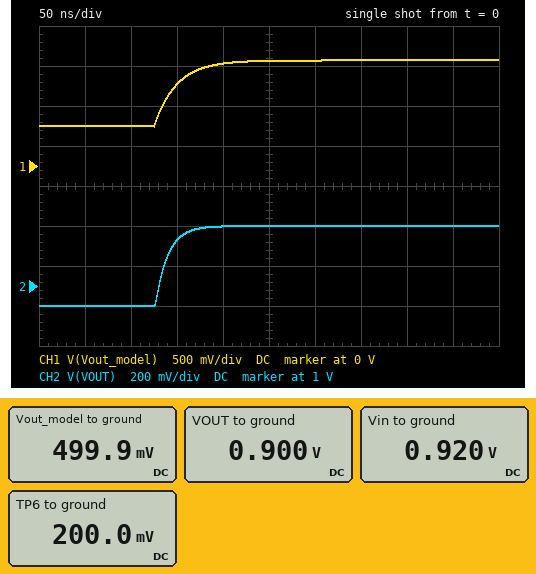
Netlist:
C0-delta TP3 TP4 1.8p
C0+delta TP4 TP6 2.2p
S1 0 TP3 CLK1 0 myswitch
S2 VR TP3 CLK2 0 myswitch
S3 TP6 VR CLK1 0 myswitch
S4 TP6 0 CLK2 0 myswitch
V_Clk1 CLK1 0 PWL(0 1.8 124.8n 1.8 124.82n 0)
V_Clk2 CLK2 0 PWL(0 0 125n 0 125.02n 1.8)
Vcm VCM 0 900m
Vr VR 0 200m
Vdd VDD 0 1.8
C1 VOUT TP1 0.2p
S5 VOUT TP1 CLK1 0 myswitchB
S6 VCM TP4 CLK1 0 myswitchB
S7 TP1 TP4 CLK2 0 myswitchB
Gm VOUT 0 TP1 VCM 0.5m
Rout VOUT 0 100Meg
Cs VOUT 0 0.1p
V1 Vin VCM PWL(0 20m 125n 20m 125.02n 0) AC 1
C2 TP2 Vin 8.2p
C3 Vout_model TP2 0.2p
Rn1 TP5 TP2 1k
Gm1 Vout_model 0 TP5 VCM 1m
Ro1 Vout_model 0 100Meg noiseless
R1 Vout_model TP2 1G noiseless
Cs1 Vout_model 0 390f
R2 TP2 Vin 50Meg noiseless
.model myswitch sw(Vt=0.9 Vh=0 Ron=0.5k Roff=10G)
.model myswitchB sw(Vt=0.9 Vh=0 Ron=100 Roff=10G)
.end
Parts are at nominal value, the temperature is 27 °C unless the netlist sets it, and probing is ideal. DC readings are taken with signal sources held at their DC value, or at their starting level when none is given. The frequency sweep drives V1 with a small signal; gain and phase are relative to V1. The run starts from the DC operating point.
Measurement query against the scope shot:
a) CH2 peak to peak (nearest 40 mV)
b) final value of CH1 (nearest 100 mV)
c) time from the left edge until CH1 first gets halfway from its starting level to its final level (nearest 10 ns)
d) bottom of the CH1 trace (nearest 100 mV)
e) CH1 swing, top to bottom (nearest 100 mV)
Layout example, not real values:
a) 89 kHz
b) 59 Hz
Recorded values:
a) 400 mV
b) 1.3 V
c) 140 ns
d) 500 mV
e) 800 mV
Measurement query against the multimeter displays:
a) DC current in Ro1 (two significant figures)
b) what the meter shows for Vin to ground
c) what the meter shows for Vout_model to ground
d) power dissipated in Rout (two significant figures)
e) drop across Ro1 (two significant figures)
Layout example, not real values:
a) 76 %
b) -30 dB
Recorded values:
a) 5.0 nA
b) 0.920 V
c) 499.9 mV
d) 8.1 nW
e) 500 mV
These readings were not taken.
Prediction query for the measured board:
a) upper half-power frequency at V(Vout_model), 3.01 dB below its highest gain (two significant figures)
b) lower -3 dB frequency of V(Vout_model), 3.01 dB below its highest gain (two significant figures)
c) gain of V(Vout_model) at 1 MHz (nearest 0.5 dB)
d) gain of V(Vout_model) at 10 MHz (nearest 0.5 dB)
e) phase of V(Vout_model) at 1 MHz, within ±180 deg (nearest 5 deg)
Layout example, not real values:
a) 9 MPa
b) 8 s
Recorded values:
a) 6.5 MHz
b) 580 Hz
c) 32.0 dB
d) 27.0 dB
e) 170 deg
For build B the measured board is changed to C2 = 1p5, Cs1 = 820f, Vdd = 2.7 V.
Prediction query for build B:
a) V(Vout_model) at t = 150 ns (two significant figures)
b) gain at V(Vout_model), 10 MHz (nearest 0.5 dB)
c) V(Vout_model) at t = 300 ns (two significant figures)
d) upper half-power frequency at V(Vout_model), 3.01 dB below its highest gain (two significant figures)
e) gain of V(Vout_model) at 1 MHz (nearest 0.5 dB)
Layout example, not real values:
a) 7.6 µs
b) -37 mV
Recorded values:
a) 640 mV
b) 16.5 dB
c) 650 mV
d) 940 Hz
e) 17.5 dB
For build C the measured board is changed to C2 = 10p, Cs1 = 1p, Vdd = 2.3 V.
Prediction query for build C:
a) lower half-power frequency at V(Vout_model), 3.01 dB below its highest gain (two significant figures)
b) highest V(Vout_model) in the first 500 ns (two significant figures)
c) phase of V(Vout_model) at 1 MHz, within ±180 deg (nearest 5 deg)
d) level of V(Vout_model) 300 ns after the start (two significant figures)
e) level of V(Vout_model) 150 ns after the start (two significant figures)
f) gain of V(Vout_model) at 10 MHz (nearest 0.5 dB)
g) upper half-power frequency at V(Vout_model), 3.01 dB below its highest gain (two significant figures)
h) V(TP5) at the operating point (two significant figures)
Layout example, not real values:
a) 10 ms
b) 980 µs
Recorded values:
a) 660 Hz
b) 1.5 V
c) 160 deg
d) 1.4 V
e) 830 mV
f) 22.0 dB
g) 2.6 MHz
h) 900 mV
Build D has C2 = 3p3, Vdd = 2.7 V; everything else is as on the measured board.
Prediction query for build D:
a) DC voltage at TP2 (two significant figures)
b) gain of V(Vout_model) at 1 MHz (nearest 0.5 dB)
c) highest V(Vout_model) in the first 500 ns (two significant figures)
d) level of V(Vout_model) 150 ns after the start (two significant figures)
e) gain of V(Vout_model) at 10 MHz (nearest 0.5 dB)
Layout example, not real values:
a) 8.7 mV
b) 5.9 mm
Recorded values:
a) 900 mV
b) 24.5 dB
c) 830 mV
d) 800 mV
e) 23.0 dB
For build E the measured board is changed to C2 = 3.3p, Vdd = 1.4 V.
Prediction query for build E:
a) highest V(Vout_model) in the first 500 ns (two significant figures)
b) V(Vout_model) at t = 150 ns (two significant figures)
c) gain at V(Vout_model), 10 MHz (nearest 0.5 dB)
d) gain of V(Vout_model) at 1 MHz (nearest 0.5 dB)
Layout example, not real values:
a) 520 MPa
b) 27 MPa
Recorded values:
a) 830 mV
b) 800 mV
c) 23.0 dB
d) 24.5 dB
